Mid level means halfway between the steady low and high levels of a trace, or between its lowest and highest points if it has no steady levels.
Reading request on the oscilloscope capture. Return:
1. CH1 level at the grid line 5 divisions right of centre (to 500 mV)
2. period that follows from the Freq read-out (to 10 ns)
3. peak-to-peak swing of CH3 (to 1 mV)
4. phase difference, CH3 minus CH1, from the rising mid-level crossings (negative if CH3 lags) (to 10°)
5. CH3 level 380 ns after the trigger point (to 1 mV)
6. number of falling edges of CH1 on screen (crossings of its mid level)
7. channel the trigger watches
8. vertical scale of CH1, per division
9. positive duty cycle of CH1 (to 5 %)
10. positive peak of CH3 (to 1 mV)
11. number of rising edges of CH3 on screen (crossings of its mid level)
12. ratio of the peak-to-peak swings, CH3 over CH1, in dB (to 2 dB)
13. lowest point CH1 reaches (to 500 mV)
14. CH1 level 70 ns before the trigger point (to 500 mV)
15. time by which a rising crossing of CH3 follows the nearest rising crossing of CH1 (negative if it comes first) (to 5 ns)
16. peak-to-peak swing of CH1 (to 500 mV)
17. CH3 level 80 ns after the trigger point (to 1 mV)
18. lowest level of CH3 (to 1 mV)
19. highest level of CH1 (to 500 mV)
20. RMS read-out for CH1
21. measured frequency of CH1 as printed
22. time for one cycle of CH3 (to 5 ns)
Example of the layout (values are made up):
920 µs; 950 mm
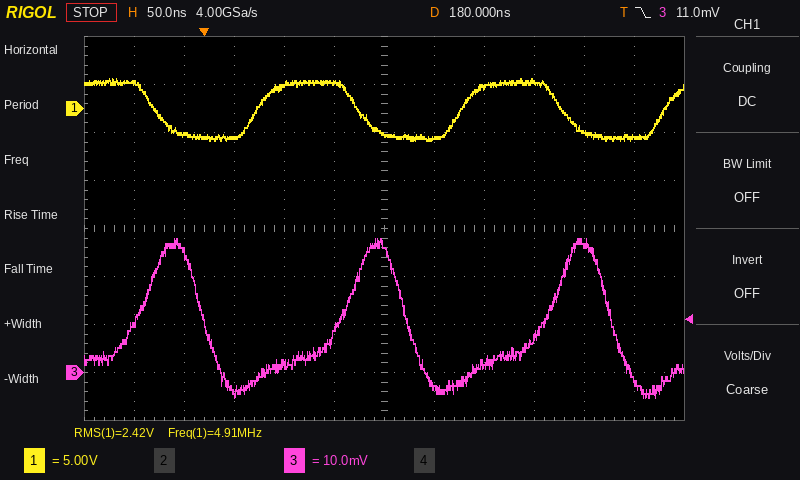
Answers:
-3.0 V; 200 ns; 33 mV; -150°; 27 mV; 3; CH3; 5 V; 50 %; 28 mV; 3; -46 dB; -3.5 V; 2.5 V; +85 ns; 6.5 V; 2 mV; -5 mV; 3.0 V; 2.42 V; 4.91 MHz; 205 ns
